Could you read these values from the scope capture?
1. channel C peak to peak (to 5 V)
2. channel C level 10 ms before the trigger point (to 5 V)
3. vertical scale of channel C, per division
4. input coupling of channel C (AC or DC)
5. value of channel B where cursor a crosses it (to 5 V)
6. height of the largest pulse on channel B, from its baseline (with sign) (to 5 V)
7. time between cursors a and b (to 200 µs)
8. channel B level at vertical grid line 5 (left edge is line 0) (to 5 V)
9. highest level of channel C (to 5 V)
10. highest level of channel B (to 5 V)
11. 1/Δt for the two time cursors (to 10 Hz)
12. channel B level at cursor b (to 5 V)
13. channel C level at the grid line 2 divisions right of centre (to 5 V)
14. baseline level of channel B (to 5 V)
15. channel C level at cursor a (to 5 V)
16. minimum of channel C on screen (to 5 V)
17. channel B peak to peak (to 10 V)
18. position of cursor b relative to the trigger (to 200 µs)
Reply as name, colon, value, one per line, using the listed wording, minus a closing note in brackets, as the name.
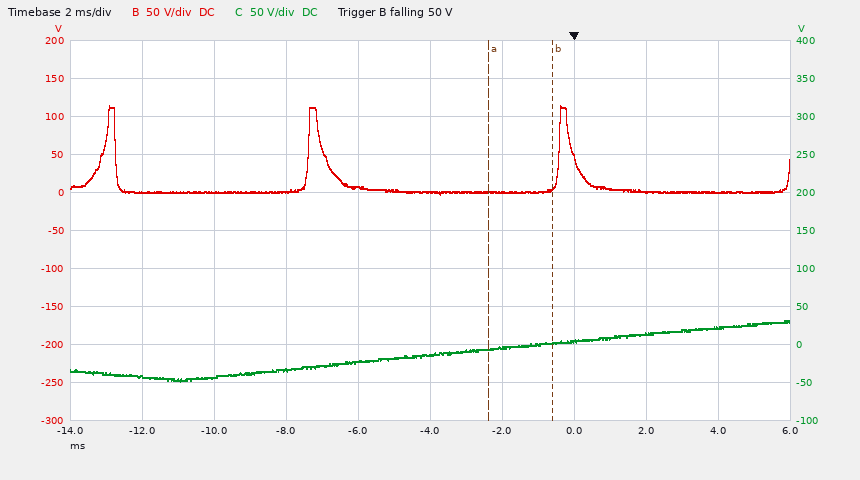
channel C peak to peak: 80 V
channel C level 10 ms before the trigger point: -45 V
vertical scale of channel C, per division: 50 V
input coupling of channel C: DC
value of channel B where cursor a crosses it: 0 V
height of the largest pulse on channel B, from its baseline (with sign): +115 V
time between cursors a and b: 1.8 ms
channel B level at vertical grid line 5 (left edge is line 0): 0 V
highest level of channel C: 30 V
highest level of channel B: 115 V
1/Δt for the two time cursors: 560 Hz
channel B level at cursor b: 5 V
channel C level at the grid line 2 divisions right of centre: 5 V
baseline level of channel B: 0 V
channel C level at cursor a: -5 V
minimum of channel C on screen: -50 V
channel B peak to peak: 120 V
position of cursor b relative to the trigger: -600 µs
